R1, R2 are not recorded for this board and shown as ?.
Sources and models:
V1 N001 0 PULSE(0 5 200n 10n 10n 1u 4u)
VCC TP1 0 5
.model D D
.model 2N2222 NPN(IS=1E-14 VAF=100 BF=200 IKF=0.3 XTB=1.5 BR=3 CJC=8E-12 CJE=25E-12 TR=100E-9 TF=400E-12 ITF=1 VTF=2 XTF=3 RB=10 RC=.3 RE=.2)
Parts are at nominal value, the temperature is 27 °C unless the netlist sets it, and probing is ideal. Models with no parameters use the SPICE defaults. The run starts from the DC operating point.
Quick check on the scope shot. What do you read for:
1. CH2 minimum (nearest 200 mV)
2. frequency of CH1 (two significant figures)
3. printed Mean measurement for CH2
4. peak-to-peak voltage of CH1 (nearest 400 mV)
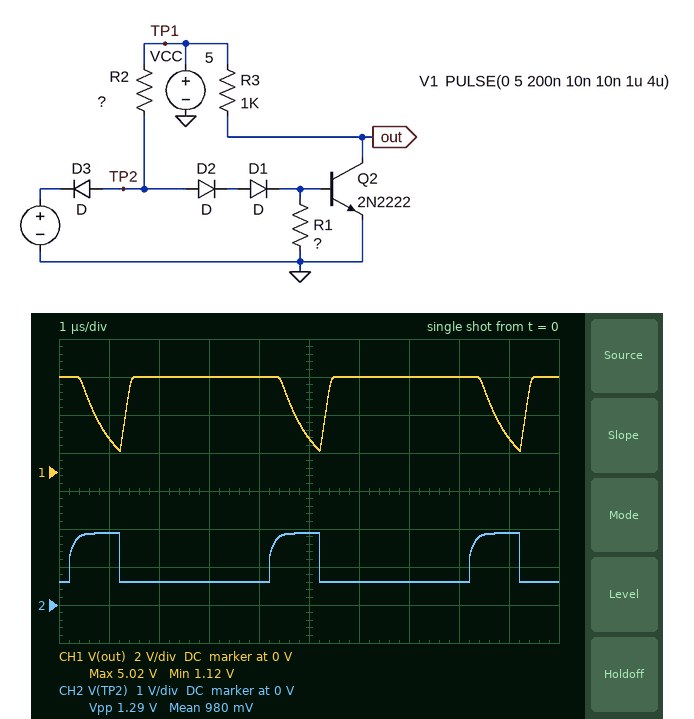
600 mV
250 kHz
980 mV
4.0 V
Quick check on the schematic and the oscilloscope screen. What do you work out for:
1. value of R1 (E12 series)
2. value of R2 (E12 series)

6.8 kΩ
22 kΩ
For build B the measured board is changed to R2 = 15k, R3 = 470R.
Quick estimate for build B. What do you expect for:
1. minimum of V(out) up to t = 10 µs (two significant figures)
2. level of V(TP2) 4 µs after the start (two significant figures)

130 mV
620 mV
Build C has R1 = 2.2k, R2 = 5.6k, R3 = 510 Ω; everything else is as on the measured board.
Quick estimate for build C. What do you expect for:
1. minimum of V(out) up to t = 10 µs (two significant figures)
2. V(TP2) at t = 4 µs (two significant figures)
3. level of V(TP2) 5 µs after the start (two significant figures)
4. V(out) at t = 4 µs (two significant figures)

87 mV
650 mV
2.0 V
5.0 V
